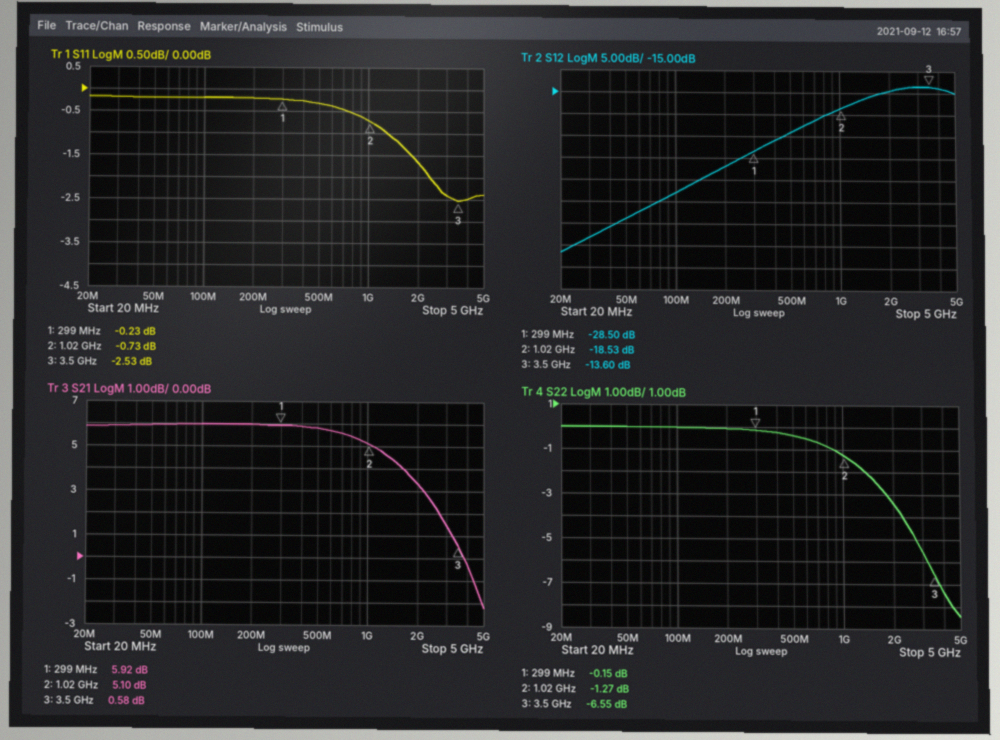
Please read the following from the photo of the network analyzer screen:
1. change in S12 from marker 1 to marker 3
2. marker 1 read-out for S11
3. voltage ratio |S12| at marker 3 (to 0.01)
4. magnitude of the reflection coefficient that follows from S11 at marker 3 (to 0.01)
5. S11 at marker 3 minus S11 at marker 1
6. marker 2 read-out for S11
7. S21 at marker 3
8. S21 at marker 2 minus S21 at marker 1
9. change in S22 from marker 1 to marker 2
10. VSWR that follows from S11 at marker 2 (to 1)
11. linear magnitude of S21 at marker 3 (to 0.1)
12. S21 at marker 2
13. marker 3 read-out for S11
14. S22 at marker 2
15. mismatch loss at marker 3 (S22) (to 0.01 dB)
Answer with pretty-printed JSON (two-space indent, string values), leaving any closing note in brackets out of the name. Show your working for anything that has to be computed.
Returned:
{
  "change in S12 from marker 1 to marker 3": "-13.6 − (-28.5) = 14.90 dB",
  "marker 1 read-out for S11": "-0.23 dB",
  "voltage ratio |S12| at marker 3": "10^(-13.6/20) ≈ 0.21",
  "magnitude of the reflection coefficient that follows from S11 at marker 3": "10^(-2.53/20) ≈ 0.75",
  "S11 at marker 3 minus S11 at marker 1": "-2.53 − (-0.23) = -2.30 dB",
  "marker 2 read-out for S11": "-0.73 dB",
  "S21 at marker 3": "0.58 dB",
  "S21 at marker 2 minus S21 at marker 1": "5.1 − (5.92) = -0.82 dB",
  "change in S22 from marker 1 to marker 2": "-1.27 − (-0.15) = -1.12 dB",
  "VSWR that follows from S11 at marker 2": "(1 + 0.9194)/(1 − 0.9194) ≈ 24",
  "linear magnitude of S21 at marker 3": "10^(0.58/20) ≈ 1.1",
  "S21 at marker 2": "5.10 dB",
  "marker 3 read-out for S11": "-2.53 dB",
  "S22 at marker 2": "-1.27 dB",
  "mismatch loss at marker 3 (S22)": "−10 log10(1 − 10^(-6.55/10)) ≈ 1.09 dB"
}
